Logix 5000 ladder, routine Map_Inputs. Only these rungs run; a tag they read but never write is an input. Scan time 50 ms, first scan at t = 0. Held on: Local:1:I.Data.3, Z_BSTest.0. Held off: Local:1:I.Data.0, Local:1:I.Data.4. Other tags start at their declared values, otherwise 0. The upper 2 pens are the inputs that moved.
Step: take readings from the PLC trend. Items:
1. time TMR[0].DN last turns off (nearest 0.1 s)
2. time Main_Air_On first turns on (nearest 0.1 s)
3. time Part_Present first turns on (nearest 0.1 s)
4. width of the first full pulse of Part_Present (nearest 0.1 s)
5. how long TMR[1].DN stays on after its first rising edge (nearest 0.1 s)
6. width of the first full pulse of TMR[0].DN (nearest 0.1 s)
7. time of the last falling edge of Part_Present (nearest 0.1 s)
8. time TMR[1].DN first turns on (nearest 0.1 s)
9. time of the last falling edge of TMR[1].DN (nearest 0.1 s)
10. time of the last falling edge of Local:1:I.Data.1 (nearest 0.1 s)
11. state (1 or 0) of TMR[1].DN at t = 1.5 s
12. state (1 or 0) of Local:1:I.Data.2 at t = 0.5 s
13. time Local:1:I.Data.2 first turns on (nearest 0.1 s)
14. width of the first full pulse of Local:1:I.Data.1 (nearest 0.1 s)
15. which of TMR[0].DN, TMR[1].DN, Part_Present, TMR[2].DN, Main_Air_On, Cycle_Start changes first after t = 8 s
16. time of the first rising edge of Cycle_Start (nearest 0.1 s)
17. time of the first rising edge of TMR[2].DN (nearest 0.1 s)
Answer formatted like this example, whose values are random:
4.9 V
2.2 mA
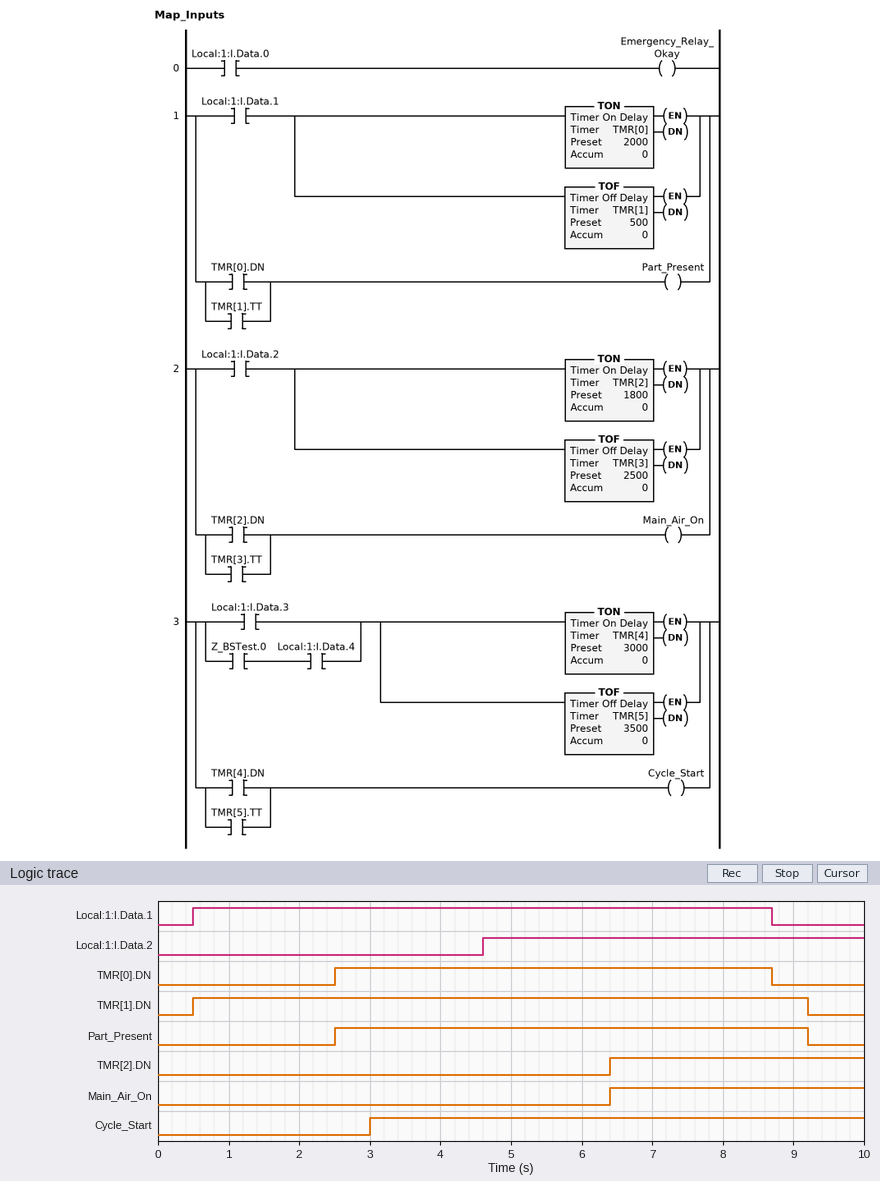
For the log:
8.7 s
6.4 s
2.5 s
6.7 s
8.7 s
6.2 s
9.2 s
0.5 s
9.2 s
8.7 s
1
0
4.6 s
8.2 s
TMR[0].DN
3.0 s
6.4 s
